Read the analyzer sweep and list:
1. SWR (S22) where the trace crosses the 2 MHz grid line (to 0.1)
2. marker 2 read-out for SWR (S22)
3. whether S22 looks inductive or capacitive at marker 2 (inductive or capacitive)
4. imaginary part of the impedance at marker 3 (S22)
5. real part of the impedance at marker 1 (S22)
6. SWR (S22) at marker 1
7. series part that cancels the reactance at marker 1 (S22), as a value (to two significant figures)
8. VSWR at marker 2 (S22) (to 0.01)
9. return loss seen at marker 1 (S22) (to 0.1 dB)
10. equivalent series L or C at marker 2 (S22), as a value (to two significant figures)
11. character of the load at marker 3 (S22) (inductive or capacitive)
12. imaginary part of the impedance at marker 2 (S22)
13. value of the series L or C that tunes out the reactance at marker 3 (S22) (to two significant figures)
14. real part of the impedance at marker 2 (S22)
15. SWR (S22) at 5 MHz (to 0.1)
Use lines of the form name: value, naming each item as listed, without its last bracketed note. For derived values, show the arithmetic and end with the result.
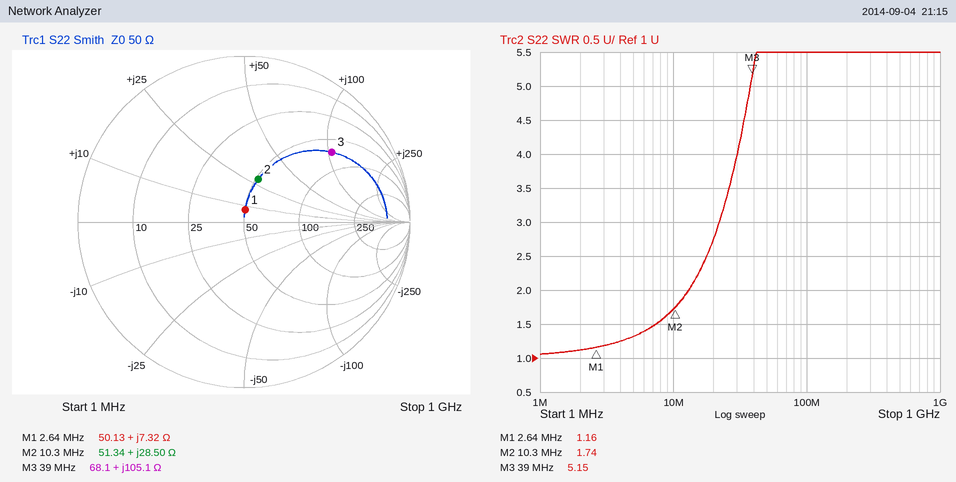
SWR (S22) where the trace crosses the 2 MHz grid line: 1.1
marker 2 read-out for SWR: 1.74
whether S22 looks inductive or capacitive at marker 2: inductive
imaginary part of the impedance at marker 3: +105.1 Ω
real part of the impedance at marker 1: 50.13 Ω
SWR (S22) at marker 1: 1.16
series part that cancels the reactance at marker 1 (S22), as a value: C = 1/(2π × 2.64 MHz × 7.32 Ω) ≈ 8.2 nF
VSWR at marker 2 (S22): 1.74
return loss seen at marker 1 (S22): 22.7 dB
equivalent series L or C at marker 2 (S22), as a value: L = 28.5 Ω/(2π × 10.3 MHz) ≈ 440 nH
character of the load at marker 3 (S22): inductive
imaginary part of the impedance at marker 2: +28.50 Ω
value of the series L or C that tunes out the reactance at marker 3 (S22): C = 1/(2π × 39 MHz × 105.1 Ω) ≈ 39 pF
real part of the impedance at marker 2: 51.34 Ω
SWR (S22) at 5 MHz: 1.3
